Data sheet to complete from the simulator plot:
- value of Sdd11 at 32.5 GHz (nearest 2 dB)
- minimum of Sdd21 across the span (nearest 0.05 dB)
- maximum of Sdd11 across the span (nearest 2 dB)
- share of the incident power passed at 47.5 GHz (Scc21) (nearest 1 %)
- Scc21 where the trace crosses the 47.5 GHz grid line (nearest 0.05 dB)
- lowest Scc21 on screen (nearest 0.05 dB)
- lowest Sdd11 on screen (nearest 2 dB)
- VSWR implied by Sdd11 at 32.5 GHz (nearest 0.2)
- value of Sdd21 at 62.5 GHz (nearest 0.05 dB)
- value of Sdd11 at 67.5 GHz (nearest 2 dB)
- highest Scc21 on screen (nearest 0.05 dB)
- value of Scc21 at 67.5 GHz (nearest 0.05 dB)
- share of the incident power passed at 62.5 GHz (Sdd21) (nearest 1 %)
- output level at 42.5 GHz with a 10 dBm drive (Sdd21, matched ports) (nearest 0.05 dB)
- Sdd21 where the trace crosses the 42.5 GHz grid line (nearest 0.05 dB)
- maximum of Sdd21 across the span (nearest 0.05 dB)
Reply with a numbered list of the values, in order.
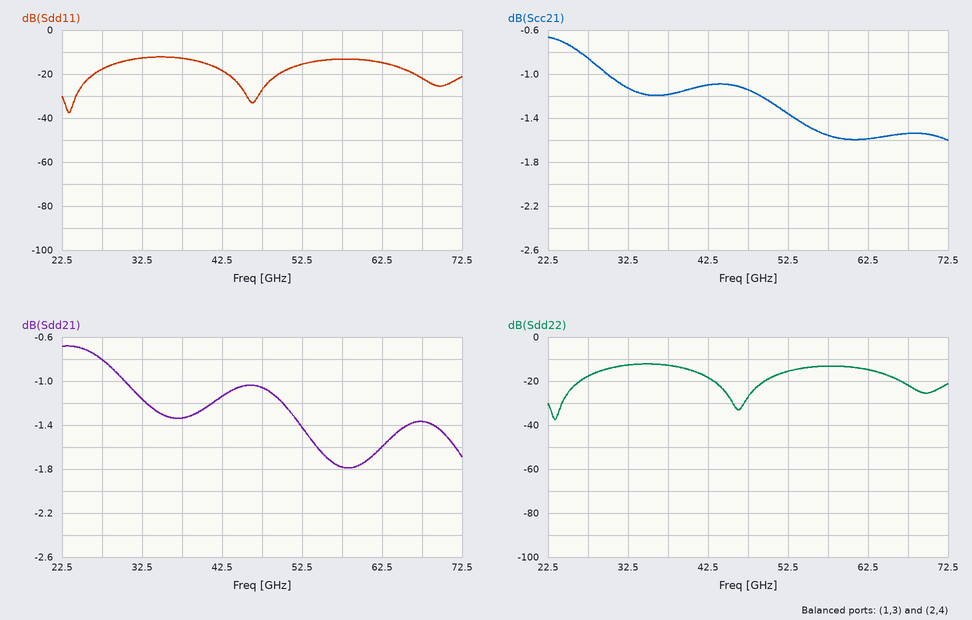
1. -12 dB
2. -1.80 dB
3. -12 dB
4. 77 %
5. -1.15 dB
6. -1.60 dB
7. -38 dB
8. 1.6
9. -1.60 dB
10. -22 dB
11. -0.65 dB
12. -1.55 dB
13. 69 %
14. 8.85 dBm
15. -1.15 dB
16. -0.70 dB
